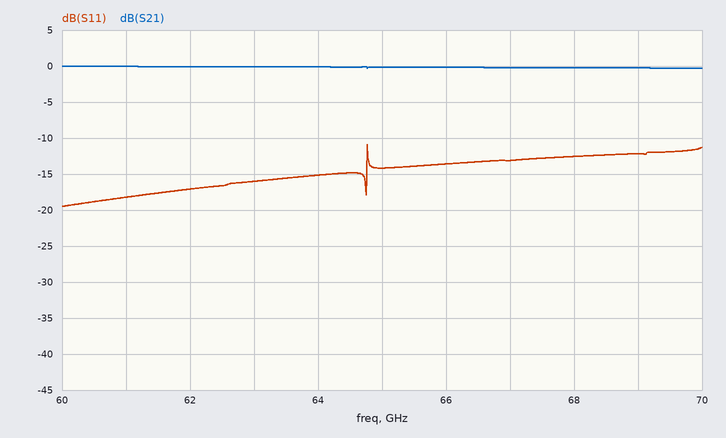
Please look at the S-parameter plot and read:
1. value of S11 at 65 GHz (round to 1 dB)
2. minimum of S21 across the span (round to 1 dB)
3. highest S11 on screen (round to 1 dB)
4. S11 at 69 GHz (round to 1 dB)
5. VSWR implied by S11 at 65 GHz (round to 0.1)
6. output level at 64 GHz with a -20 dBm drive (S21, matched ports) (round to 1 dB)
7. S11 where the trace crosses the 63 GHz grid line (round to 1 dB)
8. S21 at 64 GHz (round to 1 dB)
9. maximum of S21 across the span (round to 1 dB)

-14 dB
0 dB
-11 dB
-12 dB
1.5
-20 dBm
-16 dB
0 dB
0 dB
